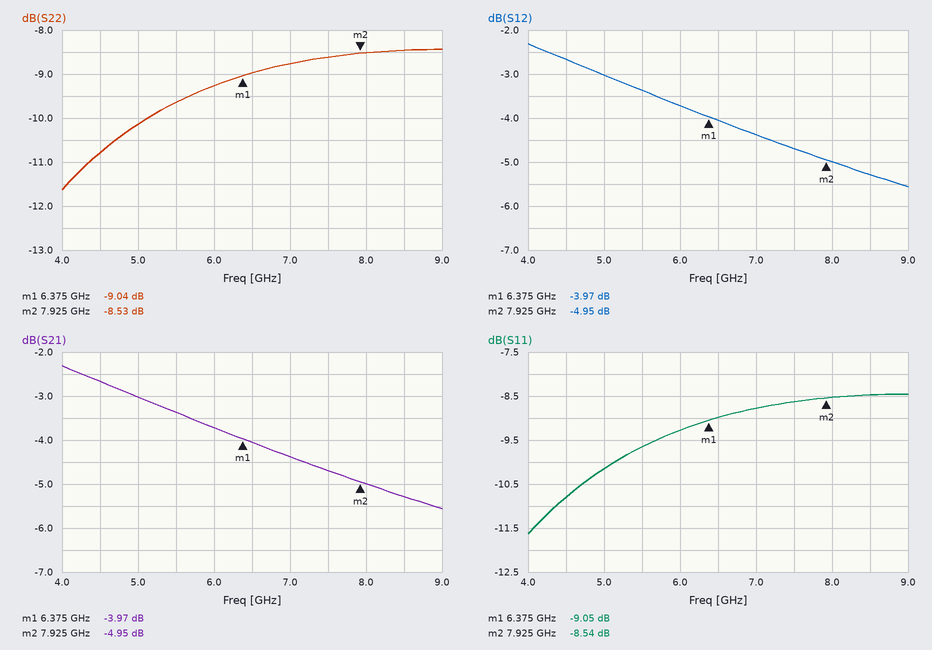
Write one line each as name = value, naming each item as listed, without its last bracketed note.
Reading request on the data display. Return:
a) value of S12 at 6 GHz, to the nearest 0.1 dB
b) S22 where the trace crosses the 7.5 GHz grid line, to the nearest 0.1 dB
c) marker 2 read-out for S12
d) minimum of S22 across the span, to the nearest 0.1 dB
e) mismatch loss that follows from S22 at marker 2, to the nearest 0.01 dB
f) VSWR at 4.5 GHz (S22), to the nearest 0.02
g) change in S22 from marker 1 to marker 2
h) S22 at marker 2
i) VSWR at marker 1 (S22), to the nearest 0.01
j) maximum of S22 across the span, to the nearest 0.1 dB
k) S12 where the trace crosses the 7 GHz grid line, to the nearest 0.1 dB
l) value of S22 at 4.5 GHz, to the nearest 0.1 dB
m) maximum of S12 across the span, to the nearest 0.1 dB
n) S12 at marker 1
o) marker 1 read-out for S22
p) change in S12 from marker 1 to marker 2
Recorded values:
value of S12 at 6 GHz, to the nearest 0.1 dB = -3.7 dB
S22 where the trace crosses the 7.5 GHz grid line, to the nearest 0.1 dB = -8.6 dB
marker 2 read-out for S12 = -4.95 dB
minimum of S22 across the span, to the nearest 0.1 dB = -11.6 dB
mismatch loss that follows from S22 at marker 2, to the nearest 0.01 dB = 0.66 dB
VSWR at 4.5 GHz (S22), to the nearest 0.02 = 1.82
change in S22 from marker 1 to marker 2 = 0.51 dB
S22 at marker 2 = -8.53 dB
VSWR at marker 1 (S22), to the nearest 0.01 = 2.09
maximum of S22 across the span, to the nearest 0.1 dB = -8.4 dB
S12 where the trace crosses the 7 GHz grid line, to the nearest 0.1 dB = -4.4 dB
value of S22 at 4.5 GHz, to the nearest 0.1 dB = -10.8 dB
maximum of S12 across the span, to the nearest 0.1 dB = -2.3 dB
S12 at marker 1 = -3.97 dB
marker 1 read-out for S22 = -9.04 dB
change in S12 from marker 1 to marker 2 = -0.98 dB
